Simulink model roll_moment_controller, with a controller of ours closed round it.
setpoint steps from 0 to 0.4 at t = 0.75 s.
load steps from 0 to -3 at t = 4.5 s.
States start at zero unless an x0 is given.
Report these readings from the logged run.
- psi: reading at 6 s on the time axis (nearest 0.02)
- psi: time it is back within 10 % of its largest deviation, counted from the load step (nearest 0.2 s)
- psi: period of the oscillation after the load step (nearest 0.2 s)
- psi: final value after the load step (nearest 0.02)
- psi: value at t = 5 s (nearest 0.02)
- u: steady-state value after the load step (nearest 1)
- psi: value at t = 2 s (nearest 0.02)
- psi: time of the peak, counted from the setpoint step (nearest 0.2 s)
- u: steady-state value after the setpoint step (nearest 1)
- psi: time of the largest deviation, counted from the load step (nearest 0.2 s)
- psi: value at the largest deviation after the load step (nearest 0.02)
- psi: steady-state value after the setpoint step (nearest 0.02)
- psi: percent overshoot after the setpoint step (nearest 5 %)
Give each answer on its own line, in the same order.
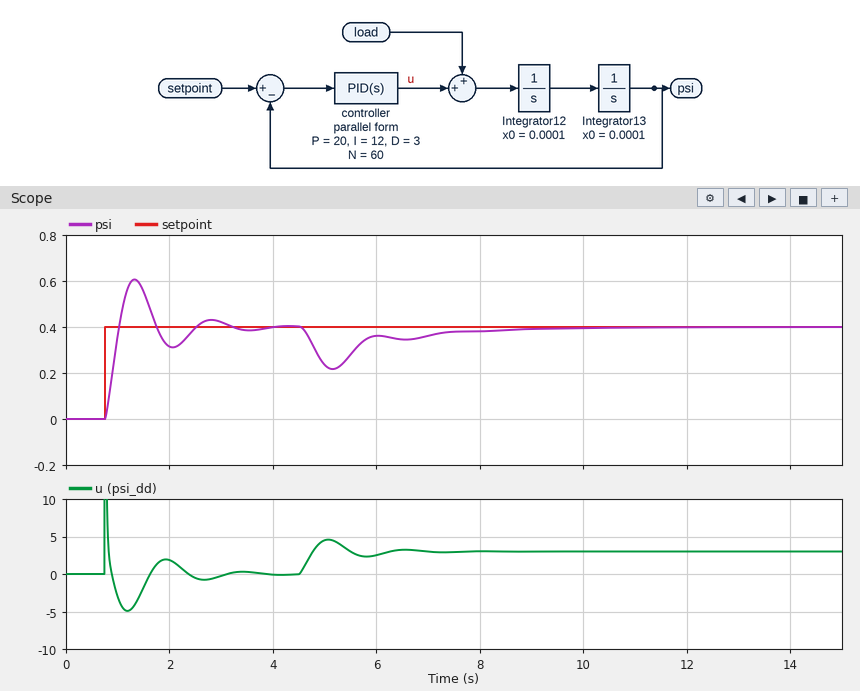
0.36
3.6 s
1.4 s
0.40
0.24
3
0.32
0.6 s
0
0.6 s
0.22
0.40
50 %
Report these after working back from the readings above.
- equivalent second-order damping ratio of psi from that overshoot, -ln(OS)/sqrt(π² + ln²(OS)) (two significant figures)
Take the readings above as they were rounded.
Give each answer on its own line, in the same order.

0.22
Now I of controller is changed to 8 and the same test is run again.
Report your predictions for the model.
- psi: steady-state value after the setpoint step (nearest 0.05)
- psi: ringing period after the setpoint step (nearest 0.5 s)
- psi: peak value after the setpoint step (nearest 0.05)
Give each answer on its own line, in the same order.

0.40
1.5 s
0.60
